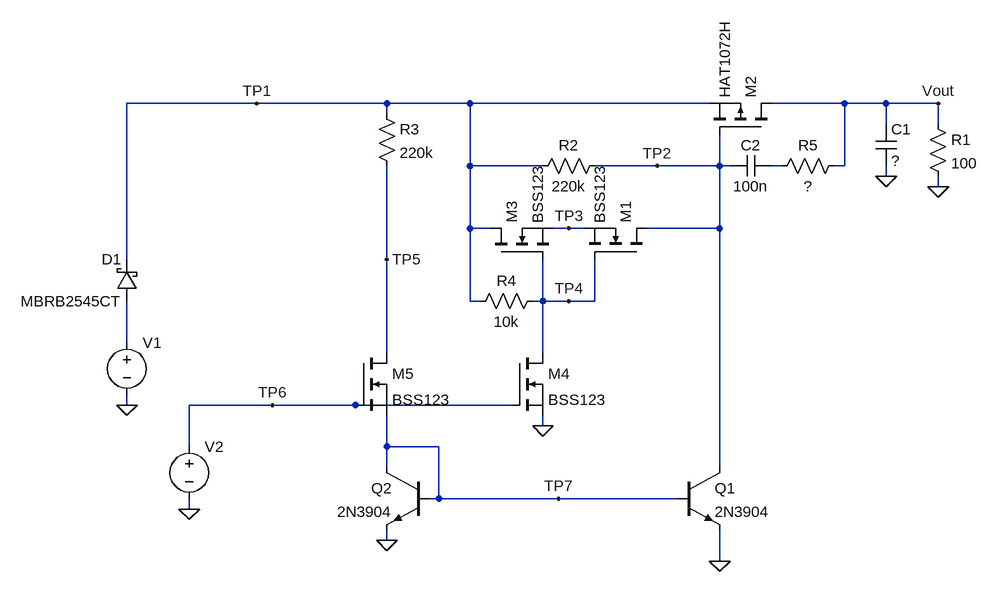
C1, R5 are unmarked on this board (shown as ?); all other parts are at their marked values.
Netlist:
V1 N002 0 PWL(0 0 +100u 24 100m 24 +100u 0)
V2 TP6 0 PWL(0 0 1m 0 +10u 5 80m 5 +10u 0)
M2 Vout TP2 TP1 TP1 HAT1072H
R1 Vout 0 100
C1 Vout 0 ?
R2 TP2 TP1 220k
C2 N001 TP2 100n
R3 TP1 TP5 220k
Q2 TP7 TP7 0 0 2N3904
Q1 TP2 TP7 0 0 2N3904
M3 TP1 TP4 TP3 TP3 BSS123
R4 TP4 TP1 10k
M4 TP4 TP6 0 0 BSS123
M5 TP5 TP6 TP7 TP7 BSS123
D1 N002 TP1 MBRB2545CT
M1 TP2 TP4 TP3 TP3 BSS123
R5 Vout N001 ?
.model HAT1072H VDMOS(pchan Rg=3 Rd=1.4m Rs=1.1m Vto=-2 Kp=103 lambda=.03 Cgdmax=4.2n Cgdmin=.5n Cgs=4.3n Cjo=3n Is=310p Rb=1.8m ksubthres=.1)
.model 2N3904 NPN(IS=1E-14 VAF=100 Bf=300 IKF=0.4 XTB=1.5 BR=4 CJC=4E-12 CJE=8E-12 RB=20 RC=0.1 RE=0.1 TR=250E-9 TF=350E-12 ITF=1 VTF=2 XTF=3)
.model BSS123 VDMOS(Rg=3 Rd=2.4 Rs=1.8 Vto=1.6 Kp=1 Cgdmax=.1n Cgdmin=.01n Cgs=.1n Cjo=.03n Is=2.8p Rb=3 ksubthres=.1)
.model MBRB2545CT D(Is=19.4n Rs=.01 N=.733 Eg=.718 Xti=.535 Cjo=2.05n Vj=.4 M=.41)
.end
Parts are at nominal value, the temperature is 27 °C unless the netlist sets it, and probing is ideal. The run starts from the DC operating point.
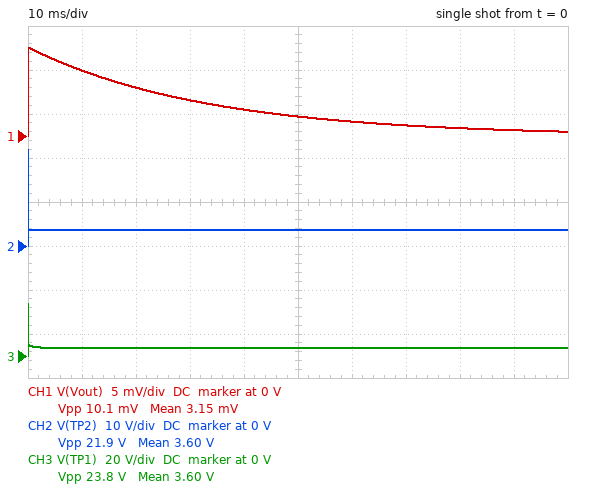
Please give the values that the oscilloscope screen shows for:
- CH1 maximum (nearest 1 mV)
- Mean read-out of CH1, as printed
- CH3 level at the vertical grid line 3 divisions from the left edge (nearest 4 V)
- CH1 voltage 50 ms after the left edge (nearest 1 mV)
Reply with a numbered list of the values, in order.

1. 10 mV
2. 3.15 mV
3. 4 V
4. 2 mV
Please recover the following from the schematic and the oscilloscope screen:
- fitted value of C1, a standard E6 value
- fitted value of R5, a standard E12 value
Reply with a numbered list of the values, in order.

1. 330 µF
2. 2.7 kΩ
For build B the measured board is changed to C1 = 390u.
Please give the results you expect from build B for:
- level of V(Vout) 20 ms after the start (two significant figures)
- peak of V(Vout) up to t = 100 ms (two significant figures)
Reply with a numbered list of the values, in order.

1. 5.1 mV
2. 8.5 mV
